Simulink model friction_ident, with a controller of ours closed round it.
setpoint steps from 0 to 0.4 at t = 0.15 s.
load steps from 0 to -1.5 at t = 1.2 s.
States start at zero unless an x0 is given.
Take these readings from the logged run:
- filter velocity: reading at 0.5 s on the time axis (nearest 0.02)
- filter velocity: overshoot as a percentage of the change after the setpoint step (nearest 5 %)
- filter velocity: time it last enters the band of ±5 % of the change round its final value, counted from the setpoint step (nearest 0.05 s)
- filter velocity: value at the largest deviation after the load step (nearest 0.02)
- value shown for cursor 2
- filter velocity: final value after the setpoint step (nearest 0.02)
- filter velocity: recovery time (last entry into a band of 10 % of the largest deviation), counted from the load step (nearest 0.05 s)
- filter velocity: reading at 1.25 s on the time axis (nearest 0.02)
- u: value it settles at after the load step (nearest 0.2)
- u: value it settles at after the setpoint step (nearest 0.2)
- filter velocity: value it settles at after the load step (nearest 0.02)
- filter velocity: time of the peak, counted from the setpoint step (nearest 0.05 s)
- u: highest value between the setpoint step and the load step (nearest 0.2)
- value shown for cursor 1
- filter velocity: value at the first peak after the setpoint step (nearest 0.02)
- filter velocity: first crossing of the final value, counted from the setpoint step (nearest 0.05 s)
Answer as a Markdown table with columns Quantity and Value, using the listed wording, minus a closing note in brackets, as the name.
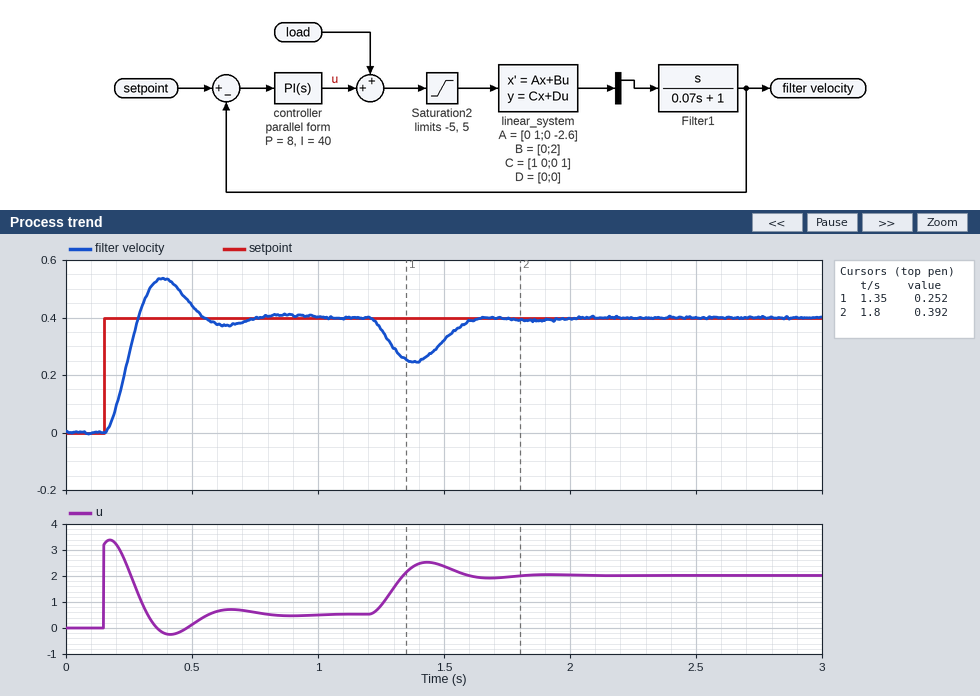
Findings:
| Quantity | Value |
|---|---|
| filter velocity: reading at 0.5 s on the time axis | 0.44 |
| filter velocity: overshoot as a percentage of the change after the setpoint step | 35 % |
| filter velocity: time it last enters the band of ±5 % of the change round its final value, counted from the setpoint step | 0.55 s |
| filter velocity: value at the largest deviation after the load step | 0.24 |
| value shown for cursor 2 | 0.392 |
| filter velocity: final value after the setpoint step | 0.40 |
| filter velocity: recovery time (last entry into a band of 10 % of the largest deviation), counted from the load step | 0.40 s |
| filter velocity: reading at 1.25 s on the time axis | 0.36 |
| u: value it settles at after the load step | 2.0 |
| u: value it settles at after the setpoint step | 0.6 |
| filter velocity: value it settles at after the load step | 0.40 |
| filter velocity: time of the peak, counted from the setpoint step | 0.25 s |
| u: highest value between the setpoint step and the load step | 3.4 |
| value shown for cursor 1 | 0.252 |
| filter velocity: value at the first peak after the setpoint step | 0.54 |
| filter velocity: first crossing of the final value, counted from the setpoint step | 0.15 s |
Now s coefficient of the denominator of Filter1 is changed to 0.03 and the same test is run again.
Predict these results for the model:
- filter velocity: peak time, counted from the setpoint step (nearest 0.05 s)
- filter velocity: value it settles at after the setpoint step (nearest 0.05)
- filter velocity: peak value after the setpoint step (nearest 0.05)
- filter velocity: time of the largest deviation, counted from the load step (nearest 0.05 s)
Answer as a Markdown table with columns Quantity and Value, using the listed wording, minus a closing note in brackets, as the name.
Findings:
| Quantity | Value |
|---|---|
| filter velocity: peak time, counted from the setpoint step | 0.20 s |
| filter velocity: value it settles at after the setpoint step | 0.40 |
| filter velocity: peak value after the setpoint step | 0.45 |
| filter velocity: time of the largest deviation, counted from the load step | 0.15 s |
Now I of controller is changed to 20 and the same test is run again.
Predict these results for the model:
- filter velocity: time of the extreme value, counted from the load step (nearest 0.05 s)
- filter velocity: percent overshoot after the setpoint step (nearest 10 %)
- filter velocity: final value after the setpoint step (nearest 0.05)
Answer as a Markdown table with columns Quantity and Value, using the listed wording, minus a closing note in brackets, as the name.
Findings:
| Quantity | Value |
|---|---|
| filter velocity: time of the extreme value, counted from the load step | 0.20 s |
| filter velocity: percent overshoot after the setpoint step | 20 % |
| filter velocity: final value after the setpoint step | 0.40 |
